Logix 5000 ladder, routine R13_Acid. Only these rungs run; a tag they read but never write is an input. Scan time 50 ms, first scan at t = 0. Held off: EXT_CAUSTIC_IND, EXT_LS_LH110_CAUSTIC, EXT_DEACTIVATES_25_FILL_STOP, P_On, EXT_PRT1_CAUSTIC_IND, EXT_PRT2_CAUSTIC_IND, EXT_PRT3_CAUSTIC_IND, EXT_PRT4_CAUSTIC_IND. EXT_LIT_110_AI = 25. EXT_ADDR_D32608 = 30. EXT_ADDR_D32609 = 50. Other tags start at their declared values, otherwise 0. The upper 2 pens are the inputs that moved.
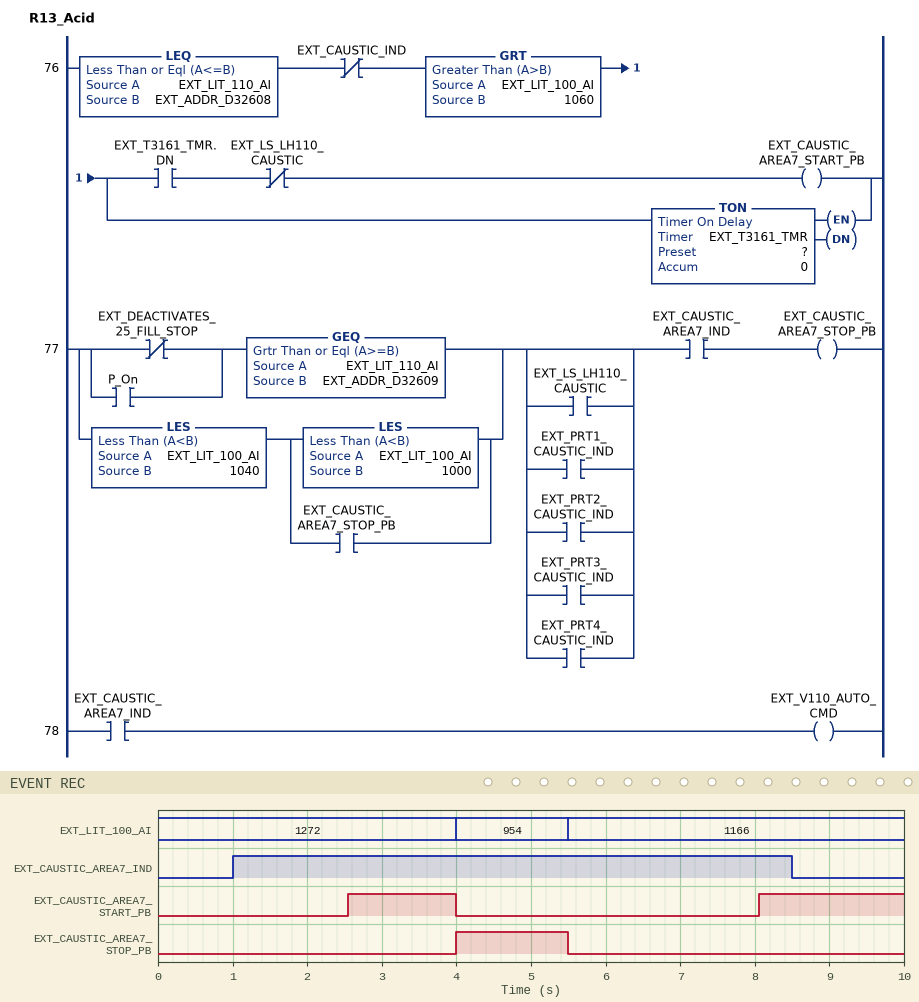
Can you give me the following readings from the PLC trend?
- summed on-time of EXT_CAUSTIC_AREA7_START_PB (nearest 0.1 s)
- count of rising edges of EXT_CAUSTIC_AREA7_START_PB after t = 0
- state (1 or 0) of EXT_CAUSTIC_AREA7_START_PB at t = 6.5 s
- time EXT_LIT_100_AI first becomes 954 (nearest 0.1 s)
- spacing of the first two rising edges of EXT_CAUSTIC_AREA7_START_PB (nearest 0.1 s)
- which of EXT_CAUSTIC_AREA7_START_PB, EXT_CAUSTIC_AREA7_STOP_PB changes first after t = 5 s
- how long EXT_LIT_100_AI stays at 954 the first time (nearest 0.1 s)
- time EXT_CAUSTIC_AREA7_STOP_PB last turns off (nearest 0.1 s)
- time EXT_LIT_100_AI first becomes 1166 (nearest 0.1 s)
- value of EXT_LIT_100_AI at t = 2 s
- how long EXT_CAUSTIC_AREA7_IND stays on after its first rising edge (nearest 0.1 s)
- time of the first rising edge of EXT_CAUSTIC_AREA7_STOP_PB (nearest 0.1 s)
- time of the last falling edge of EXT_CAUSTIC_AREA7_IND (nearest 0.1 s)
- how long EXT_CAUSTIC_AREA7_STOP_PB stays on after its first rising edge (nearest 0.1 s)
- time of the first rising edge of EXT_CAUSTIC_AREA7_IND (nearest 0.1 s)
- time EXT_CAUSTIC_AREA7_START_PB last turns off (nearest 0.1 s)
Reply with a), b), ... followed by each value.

a) 3.4 s
b) 2
c) 0
d) 4.0 s
e) 5.5 s
f) EXT_CAUSTIC_AREA7_STOP_PB
g) 1.5 s
h) 5.5 s
i) 5.5 s
j) 1272
k) 7.5 s
l) 4.0 s
m) 8.5 s
n) 1.5 s
o) 1.0 s
p) 4.0 s
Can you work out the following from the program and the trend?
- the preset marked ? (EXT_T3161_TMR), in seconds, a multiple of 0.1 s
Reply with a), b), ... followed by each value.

a) 2.5 s
